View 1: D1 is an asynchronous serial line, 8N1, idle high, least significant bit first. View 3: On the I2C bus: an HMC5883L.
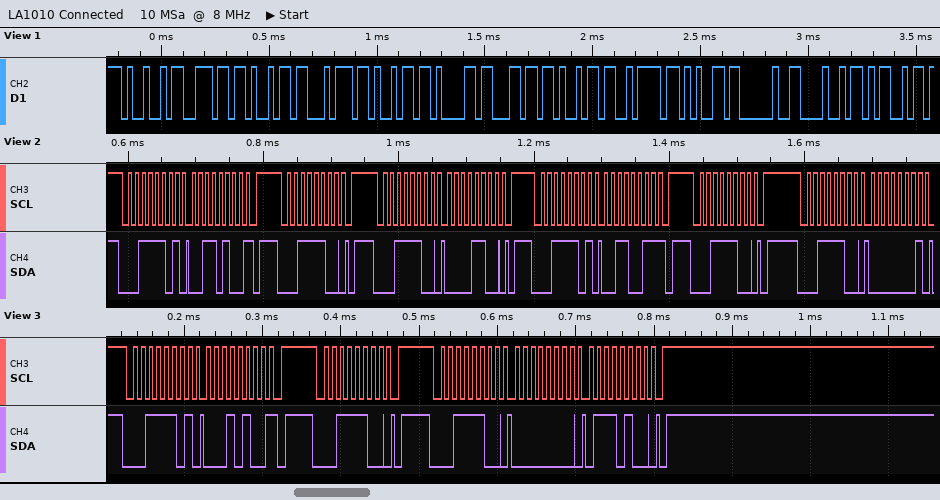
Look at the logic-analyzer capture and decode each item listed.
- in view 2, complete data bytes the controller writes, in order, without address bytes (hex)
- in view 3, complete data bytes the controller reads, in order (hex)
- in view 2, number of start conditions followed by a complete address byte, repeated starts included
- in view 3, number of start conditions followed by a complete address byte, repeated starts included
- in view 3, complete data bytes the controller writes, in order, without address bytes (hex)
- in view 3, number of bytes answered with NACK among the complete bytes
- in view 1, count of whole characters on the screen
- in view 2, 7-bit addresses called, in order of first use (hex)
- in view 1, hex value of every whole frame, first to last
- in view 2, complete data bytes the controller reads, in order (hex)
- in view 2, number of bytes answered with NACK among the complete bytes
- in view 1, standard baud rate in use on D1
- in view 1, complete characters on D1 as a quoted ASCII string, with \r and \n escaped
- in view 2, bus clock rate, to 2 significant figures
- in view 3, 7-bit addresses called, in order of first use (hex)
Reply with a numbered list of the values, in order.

1. 0C 01
2. 14
3. 6
4. 3
5. 00 74
6. 1
7. 13
8. 0x1E
9. 49 6E 69 74 69 61 6C 69 7A 65 20 48 4D
10. 34 33
11. 2
12. 38400 baud
13. "Initialize HM"
14. 100 kHz
15. 0x1E
